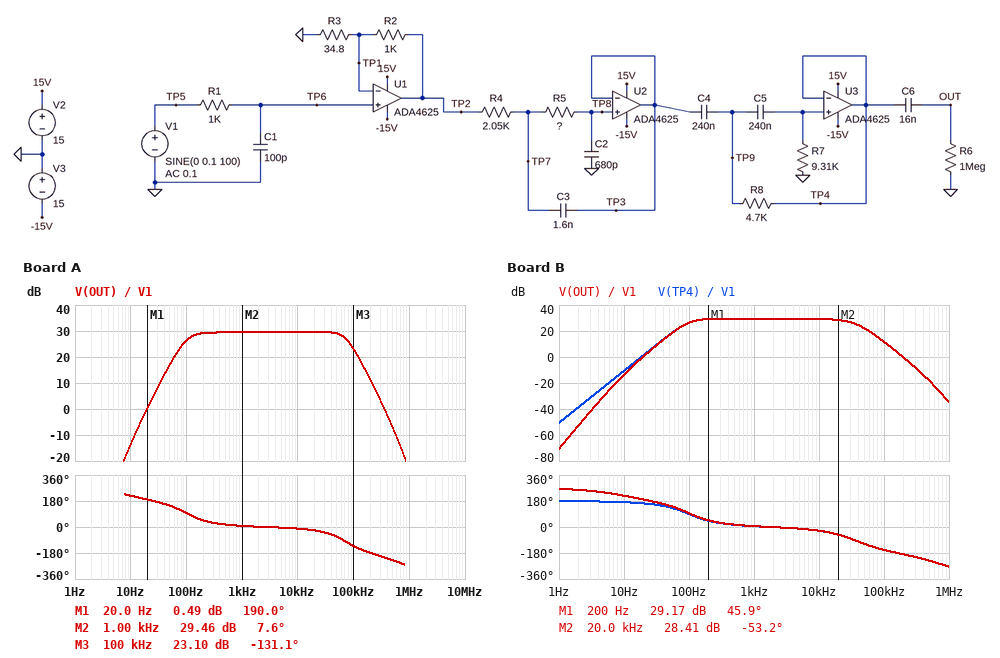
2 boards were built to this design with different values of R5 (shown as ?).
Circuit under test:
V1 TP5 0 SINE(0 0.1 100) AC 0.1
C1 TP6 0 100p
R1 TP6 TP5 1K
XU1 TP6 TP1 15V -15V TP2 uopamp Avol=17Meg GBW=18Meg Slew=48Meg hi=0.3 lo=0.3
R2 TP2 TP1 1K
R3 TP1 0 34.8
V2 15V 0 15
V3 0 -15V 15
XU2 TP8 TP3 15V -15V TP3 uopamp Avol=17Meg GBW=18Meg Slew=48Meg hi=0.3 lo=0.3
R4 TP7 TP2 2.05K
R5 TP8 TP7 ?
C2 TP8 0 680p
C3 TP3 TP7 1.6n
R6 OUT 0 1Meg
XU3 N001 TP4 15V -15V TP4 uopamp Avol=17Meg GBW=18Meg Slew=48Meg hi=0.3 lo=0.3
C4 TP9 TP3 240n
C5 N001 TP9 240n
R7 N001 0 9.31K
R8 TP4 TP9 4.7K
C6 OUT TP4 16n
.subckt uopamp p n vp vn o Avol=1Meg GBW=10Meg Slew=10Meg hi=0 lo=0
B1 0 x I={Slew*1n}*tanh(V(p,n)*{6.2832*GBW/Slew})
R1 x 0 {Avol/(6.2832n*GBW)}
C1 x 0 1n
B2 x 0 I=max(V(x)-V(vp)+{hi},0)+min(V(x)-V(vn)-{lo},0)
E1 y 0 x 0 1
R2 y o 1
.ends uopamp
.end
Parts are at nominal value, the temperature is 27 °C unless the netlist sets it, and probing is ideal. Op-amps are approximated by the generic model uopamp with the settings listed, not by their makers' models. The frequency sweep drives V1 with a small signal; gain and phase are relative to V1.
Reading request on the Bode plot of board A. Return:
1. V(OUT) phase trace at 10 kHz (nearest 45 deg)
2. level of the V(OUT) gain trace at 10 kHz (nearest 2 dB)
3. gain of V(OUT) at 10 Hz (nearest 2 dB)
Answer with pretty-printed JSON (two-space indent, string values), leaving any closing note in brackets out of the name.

{
  "V(OUT) phase trace at 10 kHz": "0 deg",
  "level of the V(OUT) gain trace at 10 kHz": "30 dB",
  "gain of V(OUT) at 10 Hz": "-14 dB"
}
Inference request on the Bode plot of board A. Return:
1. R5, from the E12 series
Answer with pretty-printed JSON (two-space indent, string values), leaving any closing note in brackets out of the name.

{
  "R5, from the E12 series": "2.2 kΩ"
}
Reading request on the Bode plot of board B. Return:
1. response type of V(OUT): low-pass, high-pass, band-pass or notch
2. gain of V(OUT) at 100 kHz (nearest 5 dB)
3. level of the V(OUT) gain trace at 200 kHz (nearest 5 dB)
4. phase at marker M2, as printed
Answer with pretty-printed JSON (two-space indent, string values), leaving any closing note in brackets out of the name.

{
  "response type of V(OUT): low-pass, high-pass, band-pass or notch": "band-pass",
  "gain of V(OUT) at 100 kHz": "10 dB",
  "level of the V(OUT) gain trace at 200 kHz": "0 dB",
  "phase at marker M2, as printed": "-53.2 deg"
}
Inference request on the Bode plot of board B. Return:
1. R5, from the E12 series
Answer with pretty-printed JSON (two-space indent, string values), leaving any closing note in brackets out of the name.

{
  "R5, from the E12 series": "8.2 kΩ"
}
